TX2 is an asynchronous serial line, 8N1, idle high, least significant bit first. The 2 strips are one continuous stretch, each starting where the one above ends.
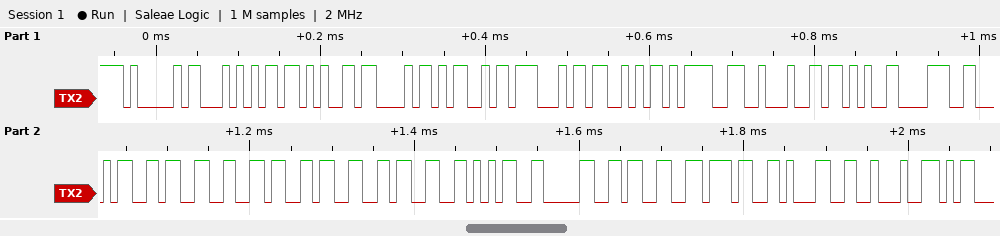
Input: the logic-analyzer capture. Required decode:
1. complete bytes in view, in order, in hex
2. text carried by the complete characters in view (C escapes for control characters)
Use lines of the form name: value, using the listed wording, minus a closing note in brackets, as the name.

complete bytes in view, in order, in hex: 0x41 0x54 0x2B 0x43 0x4D 0x47 0x53 0x3D 0x22 0x2B 0x38 0x34 0x33 0x36 0x33 0x33 0x35 0x30 0x33 0x37 0x31 0x22
text carried by the complete characters in view: "AT+CMGS=\"+84363350371\""
